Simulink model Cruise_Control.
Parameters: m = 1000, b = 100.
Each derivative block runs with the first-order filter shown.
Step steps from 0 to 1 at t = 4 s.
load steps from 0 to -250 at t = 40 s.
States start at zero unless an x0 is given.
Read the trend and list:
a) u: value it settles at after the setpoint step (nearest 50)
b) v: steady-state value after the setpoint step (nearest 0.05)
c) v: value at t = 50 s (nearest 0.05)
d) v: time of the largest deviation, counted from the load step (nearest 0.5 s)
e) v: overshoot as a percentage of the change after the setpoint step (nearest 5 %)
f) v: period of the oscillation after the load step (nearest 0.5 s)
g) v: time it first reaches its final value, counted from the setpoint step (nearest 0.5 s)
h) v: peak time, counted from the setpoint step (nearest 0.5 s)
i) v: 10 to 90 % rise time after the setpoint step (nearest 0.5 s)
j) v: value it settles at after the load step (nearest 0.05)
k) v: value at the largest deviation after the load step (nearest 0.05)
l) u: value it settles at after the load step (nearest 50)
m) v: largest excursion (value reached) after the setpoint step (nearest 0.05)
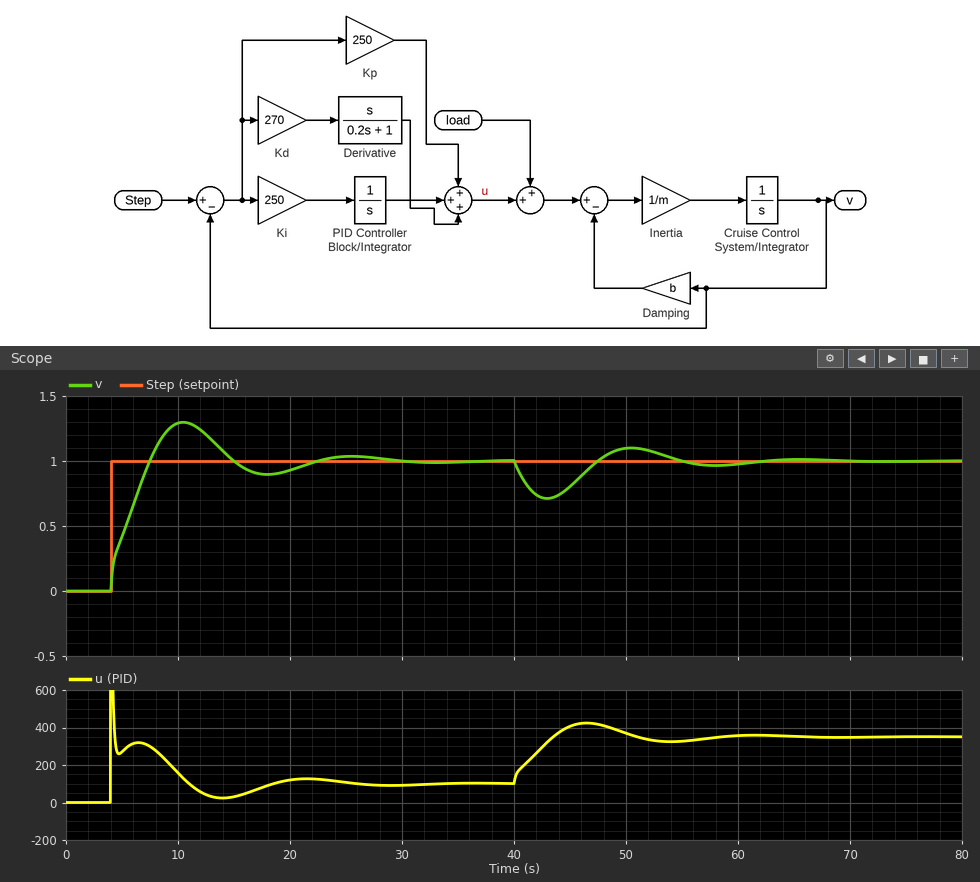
100
1.00
1.10
3.0 s
30 %
15.0 s
3.5 s
6.5 s
3.0 s
1.00
0.70
350
1.30
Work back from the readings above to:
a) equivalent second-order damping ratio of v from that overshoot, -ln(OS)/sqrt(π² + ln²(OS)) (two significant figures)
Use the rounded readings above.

0.36
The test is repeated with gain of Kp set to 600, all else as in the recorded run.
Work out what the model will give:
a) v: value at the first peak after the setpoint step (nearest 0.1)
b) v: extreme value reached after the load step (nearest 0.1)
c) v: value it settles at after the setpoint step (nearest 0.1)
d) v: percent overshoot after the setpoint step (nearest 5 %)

1.1
0.8
1.0
15 %
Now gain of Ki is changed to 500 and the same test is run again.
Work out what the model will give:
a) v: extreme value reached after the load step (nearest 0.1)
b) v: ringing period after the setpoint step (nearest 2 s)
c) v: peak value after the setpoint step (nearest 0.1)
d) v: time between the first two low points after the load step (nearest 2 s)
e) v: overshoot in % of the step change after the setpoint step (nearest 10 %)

0.8
10 s
1.4
10 s
40 %
